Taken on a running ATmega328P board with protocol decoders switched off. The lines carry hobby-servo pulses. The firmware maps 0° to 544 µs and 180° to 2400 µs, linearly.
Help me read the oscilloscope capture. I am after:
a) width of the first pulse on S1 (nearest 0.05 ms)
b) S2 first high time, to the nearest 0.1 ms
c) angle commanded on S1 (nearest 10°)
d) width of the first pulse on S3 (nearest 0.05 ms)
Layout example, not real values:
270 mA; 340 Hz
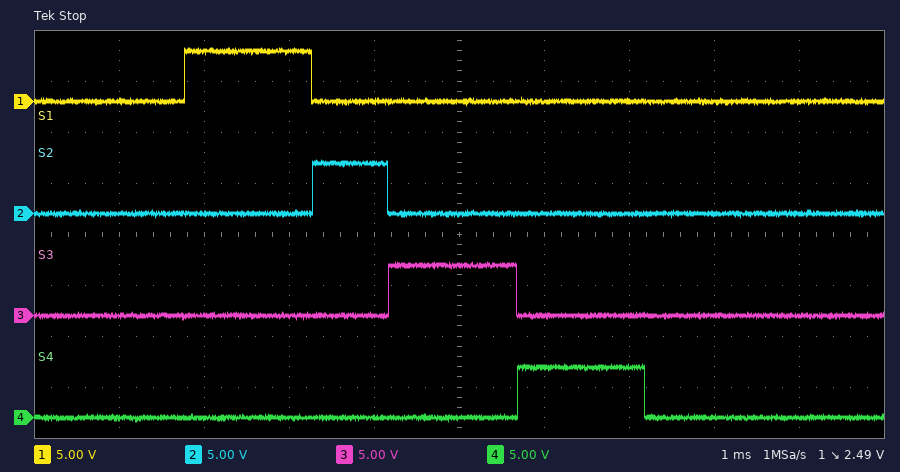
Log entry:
1.50 ms; 0.9 ms; 90°; 1.50 ms
